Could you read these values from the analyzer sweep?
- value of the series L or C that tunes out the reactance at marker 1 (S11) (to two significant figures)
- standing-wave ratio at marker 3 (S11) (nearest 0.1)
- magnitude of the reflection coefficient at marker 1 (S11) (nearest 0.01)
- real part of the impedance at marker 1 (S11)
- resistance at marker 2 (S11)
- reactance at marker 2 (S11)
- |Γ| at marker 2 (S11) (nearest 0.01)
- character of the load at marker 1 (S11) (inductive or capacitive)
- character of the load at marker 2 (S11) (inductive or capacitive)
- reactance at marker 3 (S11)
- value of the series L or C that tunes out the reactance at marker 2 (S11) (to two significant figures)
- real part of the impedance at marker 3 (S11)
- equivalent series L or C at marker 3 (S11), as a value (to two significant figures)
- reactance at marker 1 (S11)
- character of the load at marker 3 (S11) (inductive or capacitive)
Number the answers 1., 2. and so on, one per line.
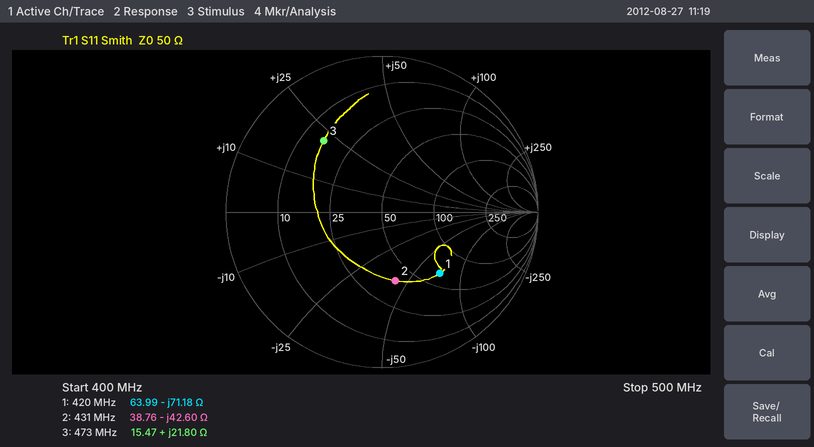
1. 27 nH
2. 3.9
3. 0.54
4. 63.99 Ω
5. 38.76 Ω
6. -42.60 Ω
7. 0.45
8. capacitive
9. capacitive
10. +21.80 Ω
11. 16 nH
12. 15.47 Ω
13. 7.3 nH
14. -71.18 Ω
15. inductive
